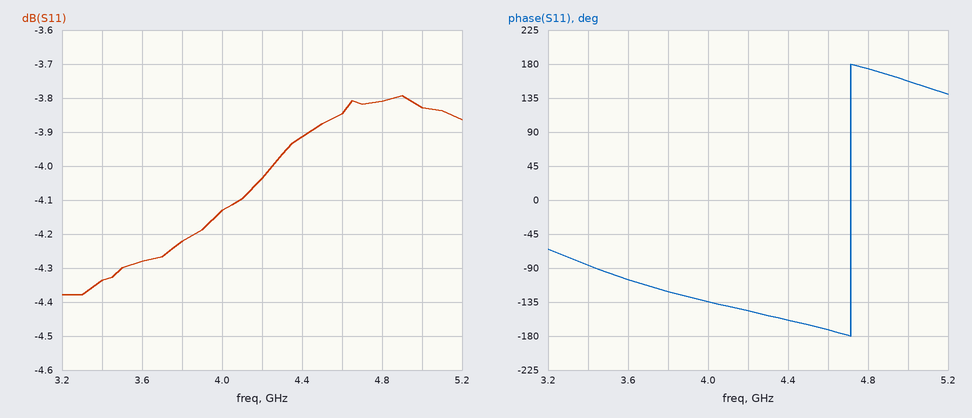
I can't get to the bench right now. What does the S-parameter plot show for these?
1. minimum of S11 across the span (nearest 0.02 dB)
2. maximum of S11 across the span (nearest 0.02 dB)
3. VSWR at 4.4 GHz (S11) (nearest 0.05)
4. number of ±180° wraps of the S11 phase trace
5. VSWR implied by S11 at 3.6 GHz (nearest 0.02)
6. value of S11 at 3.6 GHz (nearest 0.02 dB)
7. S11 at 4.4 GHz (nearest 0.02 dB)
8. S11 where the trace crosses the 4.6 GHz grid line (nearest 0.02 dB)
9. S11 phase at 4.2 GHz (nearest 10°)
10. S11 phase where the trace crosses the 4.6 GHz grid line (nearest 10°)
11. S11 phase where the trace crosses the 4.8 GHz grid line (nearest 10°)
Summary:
-4.38 dB
-3.80 dB
4.50
1
4.14
-4.28 dB
-3.92 dB
-3.84 dB
-150°
-170°
170°
